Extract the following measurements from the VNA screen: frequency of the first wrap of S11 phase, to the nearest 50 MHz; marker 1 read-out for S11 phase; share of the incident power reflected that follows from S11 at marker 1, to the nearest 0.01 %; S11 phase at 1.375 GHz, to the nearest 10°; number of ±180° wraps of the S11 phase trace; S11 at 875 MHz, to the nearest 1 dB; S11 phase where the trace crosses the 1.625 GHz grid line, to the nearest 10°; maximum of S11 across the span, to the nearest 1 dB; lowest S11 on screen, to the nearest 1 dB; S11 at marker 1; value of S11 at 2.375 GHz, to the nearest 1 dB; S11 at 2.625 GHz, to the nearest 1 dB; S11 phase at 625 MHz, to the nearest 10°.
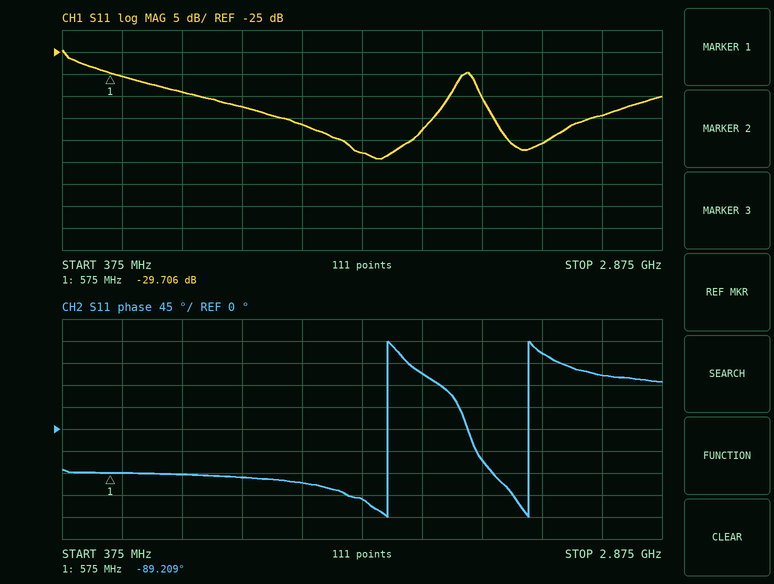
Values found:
1.75 GHz
-89.209°
0.11 %
-110°
2
-34 dB
-140°
-25 dB
-49 dB
-29.706 dB
-46 dB
-39 dB
-90°
